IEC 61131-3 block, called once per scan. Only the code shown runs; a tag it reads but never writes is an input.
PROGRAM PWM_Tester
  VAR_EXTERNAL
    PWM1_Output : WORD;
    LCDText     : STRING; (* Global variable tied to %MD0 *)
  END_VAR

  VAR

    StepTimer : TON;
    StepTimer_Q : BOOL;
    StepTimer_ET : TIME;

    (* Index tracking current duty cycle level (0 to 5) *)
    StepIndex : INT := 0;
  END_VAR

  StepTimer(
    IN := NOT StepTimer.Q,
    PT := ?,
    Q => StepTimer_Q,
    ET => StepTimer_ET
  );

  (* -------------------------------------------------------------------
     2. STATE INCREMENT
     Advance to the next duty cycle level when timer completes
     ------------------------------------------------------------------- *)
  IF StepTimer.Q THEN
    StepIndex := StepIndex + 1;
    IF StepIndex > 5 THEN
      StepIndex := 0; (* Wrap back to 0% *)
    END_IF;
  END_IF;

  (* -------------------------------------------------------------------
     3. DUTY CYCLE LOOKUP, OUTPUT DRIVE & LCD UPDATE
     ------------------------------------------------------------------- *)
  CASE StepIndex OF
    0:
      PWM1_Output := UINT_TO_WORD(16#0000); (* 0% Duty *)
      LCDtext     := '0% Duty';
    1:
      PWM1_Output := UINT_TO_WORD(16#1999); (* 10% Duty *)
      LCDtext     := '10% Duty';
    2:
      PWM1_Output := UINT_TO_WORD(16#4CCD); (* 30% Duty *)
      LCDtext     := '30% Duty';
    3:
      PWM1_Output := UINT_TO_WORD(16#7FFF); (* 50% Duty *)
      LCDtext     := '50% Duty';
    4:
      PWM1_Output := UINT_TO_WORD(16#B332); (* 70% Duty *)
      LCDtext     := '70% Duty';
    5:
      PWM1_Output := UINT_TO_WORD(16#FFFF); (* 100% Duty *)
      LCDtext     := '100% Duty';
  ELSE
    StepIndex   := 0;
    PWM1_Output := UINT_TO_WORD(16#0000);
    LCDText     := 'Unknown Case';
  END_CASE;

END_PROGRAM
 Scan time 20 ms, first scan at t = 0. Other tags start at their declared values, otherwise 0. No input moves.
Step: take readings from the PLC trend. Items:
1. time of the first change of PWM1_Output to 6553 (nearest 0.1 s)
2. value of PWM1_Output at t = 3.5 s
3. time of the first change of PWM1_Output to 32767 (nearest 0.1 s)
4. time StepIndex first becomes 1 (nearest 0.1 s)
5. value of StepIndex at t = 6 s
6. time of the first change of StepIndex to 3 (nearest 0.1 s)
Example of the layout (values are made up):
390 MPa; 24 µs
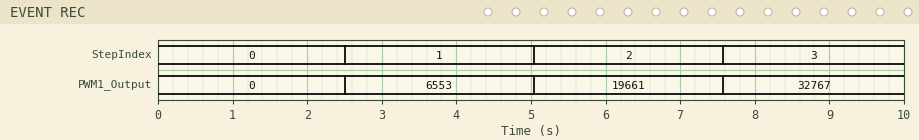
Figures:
2.5 s; 6553; 7.6 s; 2.5 s; 2; 7.6 s
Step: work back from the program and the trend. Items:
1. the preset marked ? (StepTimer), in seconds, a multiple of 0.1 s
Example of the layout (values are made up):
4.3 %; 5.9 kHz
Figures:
2.5 s
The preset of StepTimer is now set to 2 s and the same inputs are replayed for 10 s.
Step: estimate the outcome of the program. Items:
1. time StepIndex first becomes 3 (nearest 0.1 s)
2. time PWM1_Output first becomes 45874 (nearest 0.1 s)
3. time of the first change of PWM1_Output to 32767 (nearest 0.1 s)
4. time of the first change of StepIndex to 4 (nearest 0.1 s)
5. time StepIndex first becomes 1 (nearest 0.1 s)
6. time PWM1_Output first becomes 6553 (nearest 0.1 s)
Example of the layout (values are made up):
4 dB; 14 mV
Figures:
6.1 s; 8.1 s; 6.1 s; 8.1 s; 2.0 s; 2.0 s
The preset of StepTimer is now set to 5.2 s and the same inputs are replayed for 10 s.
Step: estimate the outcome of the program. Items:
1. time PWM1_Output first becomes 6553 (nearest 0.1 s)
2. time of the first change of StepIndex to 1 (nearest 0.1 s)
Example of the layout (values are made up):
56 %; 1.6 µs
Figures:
5.2 s; 5.2 s
